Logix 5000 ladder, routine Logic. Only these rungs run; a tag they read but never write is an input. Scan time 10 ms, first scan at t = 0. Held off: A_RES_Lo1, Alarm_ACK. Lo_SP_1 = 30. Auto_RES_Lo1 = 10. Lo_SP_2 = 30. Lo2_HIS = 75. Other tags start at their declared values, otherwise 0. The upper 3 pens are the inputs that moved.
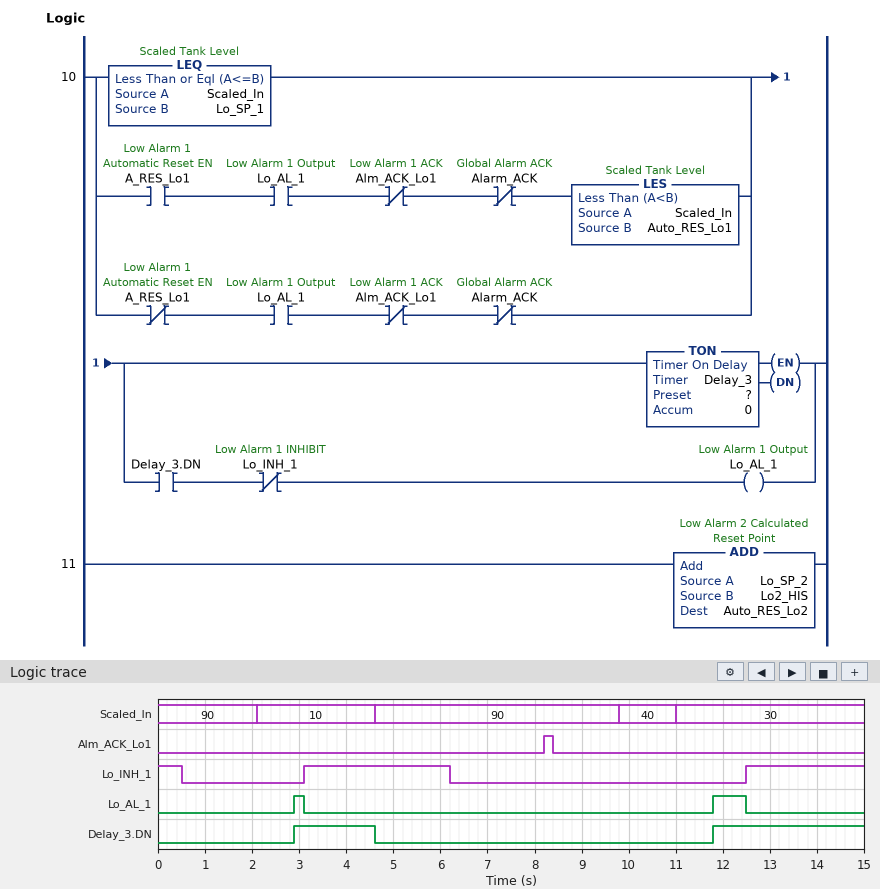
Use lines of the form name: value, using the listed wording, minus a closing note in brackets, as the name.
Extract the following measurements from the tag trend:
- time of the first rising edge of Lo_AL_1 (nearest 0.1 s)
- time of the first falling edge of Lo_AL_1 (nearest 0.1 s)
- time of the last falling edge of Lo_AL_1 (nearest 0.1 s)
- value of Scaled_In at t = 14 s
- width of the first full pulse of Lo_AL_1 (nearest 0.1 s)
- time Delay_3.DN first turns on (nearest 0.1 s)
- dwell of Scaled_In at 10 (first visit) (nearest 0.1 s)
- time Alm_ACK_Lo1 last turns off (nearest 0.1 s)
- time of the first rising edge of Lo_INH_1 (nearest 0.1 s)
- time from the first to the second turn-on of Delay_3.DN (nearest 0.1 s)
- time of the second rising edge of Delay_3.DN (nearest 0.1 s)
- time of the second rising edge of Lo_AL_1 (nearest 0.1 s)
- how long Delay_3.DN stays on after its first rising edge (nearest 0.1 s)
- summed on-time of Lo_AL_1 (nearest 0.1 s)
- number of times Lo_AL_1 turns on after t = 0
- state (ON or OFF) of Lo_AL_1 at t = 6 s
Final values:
time of the first rising edge of Lo_AL_1: 2.9 s
time of the first falling edge of Lo_AL_1: 3.1 s
time of the last falling edge of Lo_AL_1: 12.5 s
value of Scaled_In at t = 14 s: 30
width of the first full pulse of Lo_AL_1: 0.2 s
time Delay_3.DN first turns on: 2.9 s
dwell of Scaled_In at 10 (first visit): 2.5 s
time Alm_ACK_Lo1 last turns off: 8.4 s
time of the first rising edge of Lo_INH_1: 3.1 s
time from the first to the second turn-on of Delay_3.DN: 8.9 s
time of the second rising edge of Delay_3.DN: 11.8 s
time of the second rising edge of Lo_AL_1: 11.8 s
how long Delay_3.DN stays on after its first rising edge: 1.7 s
summed on-time of Lo_AL_1: 0.9 s
number of times Lo_AL_1 turns on after t = 0: 2
state (ON or OFF) of Lo_AL_1 at t = 6 s: OFF
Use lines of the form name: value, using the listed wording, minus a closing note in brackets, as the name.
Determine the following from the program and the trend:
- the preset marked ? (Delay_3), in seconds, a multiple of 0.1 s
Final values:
the preset marked ? (Delay_3), in seconds, a multiple of 0.1 s: 0.8 s
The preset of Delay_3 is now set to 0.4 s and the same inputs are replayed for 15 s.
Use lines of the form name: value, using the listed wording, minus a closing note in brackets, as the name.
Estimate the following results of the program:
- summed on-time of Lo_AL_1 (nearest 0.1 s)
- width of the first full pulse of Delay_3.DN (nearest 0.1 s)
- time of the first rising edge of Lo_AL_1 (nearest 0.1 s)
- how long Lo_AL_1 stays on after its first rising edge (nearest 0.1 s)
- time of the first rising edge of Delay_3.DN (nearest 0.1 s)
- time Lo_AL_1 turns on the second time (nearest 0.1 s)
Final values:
summed on-time of Lo_AL_1: 1.7 s
width of the first full pulse of Delay_3.DN: 2.1 s
time of the first rising edge of Lo_AL_1: 2.5 s
how long Lo_AL_1 stays on after its first rising edge: 0.6 s
time of the first rising edge of Delay_3.DN: 2.5 s
time Lo_AL_1 turns on the second time: 11.4 s
